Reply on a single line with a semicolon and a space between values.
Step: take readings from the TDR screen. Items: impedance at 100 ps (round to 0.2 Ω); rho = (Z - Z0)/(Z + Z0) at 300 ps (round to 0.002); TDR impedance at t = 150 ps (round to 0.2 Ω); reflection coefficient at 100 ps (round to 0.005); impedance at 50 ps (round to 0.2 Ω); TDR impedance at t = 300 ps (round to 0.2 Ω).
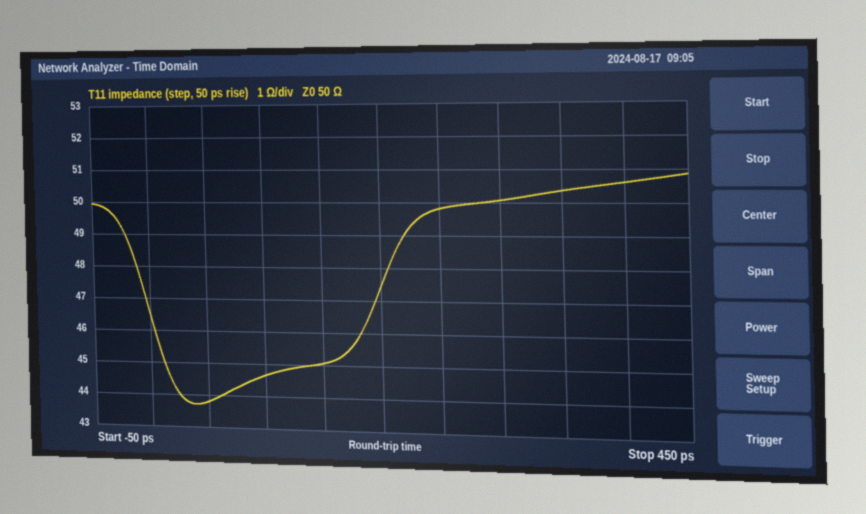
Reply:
44.6 Ω; 0.000; 45.0 Ω; -0.055; 43.8 Ω; 50.0 Ω
